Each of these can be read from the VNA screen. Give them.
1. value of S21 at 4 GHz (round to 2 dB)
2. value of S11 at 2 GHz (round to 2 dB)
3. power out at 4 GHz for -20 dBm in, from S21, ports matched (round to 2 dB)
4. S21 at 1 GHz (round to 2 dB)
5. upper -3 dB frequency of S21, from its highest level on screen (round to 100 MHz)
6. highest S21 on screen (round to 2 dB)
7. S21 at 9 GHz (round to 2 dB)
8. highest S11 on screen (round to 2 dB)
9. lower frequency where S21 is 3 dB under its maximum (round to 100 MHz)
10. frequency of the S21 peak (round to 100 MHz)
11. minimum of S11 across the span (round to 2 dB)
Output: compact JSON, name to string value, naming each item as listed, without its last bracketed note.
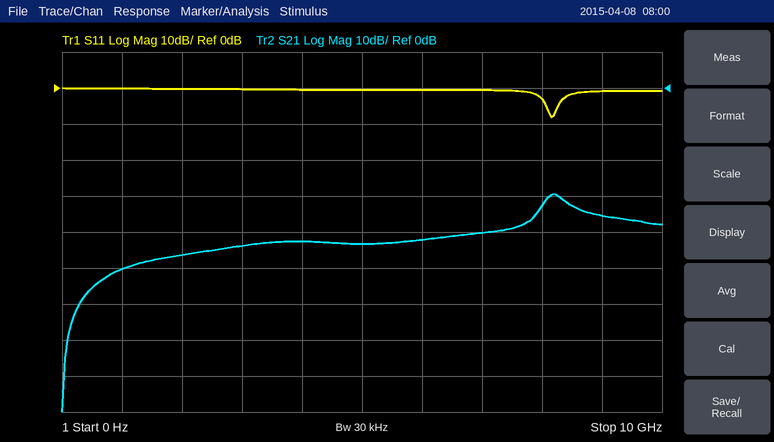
{"value of S21 at 4 GHz": "-42 dB", "value of S11 at 2 GHz": "0 dB", "power out at 4 GHz for -20 dBm in, from S21, ports matched": "-62 dBm", "S21 at 1 GHz": "-50 dB", "upper -3 dB frequency of S21, from its highest level on screen": "8.5 GHz", "highest S21 on screen": "-30 dB", "S21 at 9 GHz": "-36 dB", "highest S11 on screen": "0 dB", "lower frequency where S21 is 3 dB under its maximum": "8.0 GHz", "frequency of the S21 peak": "8.2 GHz", "minimum of S11 across the span": "-8 dB"}
